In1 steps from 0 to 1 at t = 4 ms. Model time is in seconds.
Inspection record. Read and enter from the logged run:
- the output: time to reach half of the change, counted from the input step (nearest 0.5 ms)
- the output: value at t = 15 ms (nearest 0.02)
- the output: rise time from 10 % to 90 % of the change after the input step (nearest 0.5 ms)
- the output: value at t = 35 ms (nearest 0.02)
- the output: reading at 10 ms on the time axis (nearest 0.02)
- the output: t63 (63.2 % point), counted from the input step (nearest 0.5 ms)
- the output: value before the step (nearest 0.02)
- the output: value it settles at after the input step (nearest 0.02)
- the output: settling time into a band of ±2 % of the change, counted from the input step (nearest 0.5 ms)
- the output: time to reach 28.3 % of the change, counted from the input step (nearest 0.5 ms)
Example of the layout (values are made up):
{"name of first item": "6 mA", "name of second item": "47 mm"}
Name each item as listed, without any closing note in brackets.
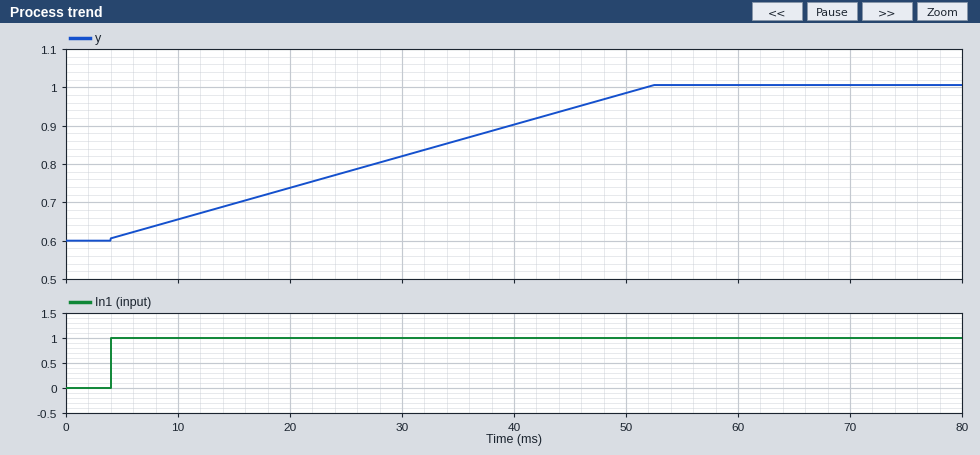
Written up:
{"the output: time to reach half of the change, counted from the input step": "24.0 ms", "the output: value at t = 15 ms": "0.70", "the output: rise time from 10 % to 90 % of the change after the input step": "39.5 ms", "the output: value at t = 35 ms": "0.86", "the output: reading at 10 ms on the time axis": "0.66", "the output: t63 (63.2 % point), counted from the input step": "30.5 ms", "the output: value before the step": "0.60", "the output: value it settles at after the input step": "1.00", "the output: settling time into a band of ±2 % of the change, counted from the input step": "47.5 ms", "the output: time to reach 28.3 % of the change, counted from the input step": "13.0 ms"}
